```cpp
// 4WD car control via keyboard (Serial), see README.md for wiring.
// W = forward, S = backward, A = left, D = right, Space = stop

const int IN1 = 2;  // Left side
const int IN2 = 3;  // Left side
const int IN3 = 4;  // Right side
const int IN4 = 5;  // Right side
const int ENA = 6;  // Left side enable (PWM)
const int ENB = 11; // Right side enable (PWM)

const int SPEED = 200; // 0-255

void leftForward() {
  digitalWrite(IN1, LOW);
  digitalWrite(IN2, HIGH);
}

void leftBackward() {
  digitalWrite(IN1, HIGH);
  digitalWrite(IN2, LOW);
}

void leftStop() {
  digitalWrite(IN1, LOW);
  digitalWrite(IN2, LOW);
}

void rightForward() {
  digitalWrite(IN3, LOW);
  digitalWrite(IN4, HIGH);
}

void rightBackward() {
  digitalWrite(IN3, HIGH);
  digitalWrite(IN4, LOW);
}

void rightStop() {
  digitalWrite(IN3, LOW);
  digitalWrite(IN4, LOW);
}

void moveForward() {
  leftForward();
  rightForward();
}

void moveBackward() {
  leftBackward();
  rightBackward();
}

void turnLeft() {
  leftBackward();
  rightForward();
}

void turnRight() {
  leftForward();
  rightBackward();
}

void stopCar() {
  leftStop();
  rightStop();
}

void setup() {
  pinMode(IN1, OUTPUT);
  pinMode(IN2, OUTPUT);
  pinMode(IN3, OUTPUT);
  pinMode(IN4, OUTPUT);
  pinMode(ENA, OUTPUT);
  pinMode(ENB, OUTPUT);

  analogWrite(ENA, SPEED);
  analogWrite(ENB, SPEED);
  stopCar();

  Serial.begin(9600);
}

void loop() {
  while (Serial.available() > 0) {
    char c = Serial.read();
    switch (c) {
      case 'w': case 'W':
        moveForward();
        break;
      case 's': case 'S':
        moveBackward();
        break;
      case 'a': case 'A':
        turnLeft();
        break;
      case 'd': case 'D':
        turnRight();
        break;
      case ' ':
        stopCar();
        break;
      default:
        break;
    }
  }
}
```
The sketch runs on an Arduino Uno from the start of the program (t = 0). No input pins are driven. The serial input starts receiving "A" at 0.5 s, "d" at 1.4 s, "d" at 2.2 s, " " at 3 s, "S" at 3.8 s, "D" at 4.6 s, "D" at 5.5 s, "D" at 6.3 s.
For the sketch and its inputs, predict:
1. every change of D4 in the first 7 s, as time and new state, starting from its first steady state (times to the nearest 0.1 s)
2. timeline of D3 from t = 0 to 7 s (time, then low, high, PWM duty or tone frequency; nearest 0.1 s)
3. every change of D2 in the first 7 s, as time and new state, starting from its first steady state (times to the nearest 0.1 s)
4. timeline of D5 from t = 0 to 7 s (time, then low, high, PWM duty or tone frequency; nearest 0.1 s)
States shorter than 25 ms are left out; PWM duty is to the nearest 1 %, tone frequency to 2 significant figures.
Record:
0 s low; 1.4 s high; 3 s low; 3.8 s high
0 s low; 1.4 s high; 3 s low; 4.6 s high
0 s low; 0.5 s high; 1.4 s low; 3.8 s high; 4.6 s low
0 s low; 0.5 s high; 1.4 s low
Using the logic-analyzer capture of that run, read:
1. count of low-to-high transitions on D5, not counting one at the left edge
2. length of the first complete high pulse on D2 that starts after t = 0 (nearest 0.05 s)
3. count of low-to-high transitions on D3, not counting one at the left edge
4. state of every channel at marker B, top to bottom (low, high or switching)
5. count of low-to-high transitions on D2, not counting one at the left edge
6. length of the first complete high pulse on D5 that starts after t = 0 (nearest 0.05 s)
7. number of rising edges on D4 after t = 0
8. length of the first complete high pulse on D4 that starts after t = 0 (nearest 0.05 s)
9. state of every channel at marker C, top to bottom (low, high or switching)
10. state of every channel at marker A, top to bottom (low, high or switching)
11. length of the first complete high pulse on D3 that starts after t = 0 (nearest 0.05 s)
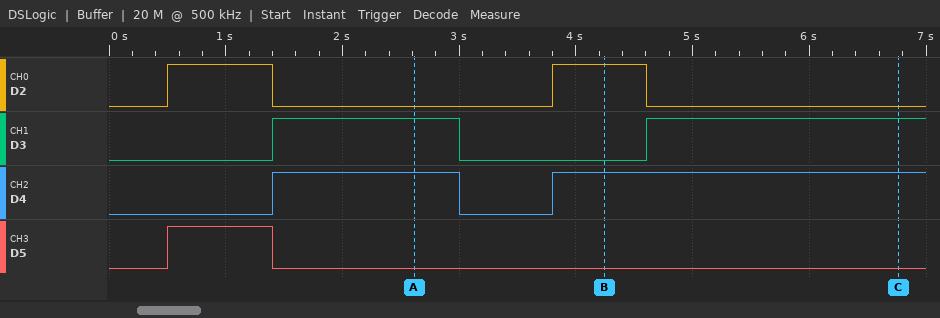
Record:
1
0.90 s
2
D2 high, D3 low, D4 high, D5 low
2
0.90 s
2
1.60 s
D2 low, D3 high, D4 high, D5 low
D2 low, D3 high, D4 high, D5 low
1.60 s
